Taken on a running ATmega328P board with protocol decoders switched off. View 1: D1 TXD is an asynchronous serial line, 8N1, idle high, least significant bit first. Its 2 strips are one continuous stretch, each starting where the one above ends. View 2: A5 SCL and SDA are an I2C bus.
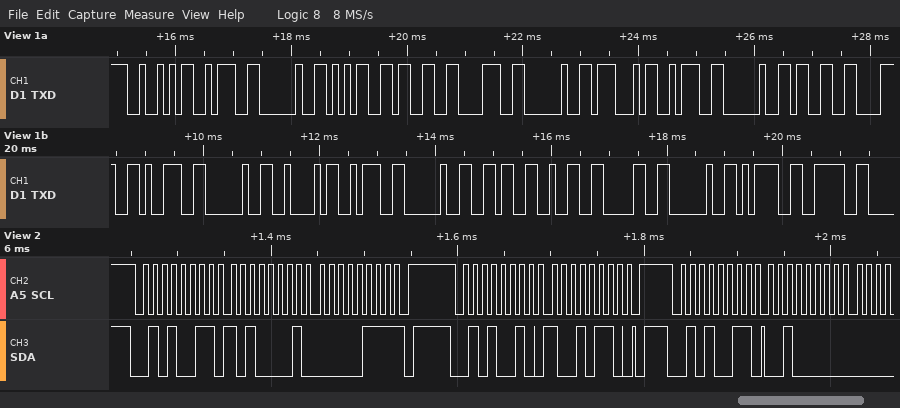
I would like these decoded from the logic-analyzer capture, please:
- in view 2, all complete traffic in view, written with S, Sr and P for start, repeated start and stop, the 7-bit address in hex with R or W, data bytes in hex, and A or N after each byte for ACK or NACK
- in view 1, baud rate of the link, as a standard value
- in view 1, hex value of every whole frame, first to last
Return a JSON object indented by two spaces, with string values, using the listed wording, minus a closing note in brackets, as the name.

{
  "in view 2, all complete traffic in view, written with S, Sr and P for start, repeated start and stop, the 7-bit address in hex with R or W, data bytes in hex, and A or N after each byte for ACK or NACK": "S 29R A A1 A 07 N P S 29W A 96 A P S 29R A 20 A",
  "in view 1, baud rate of the link, as a standard value": "9600 baud",
  "in view 1, hex value of every whole frame, first to last": "52 3A 20 35 33 38 20 47 3A 20 33 38 39 20 42 3A 20 36 32 30 20 3D 3E"
}
